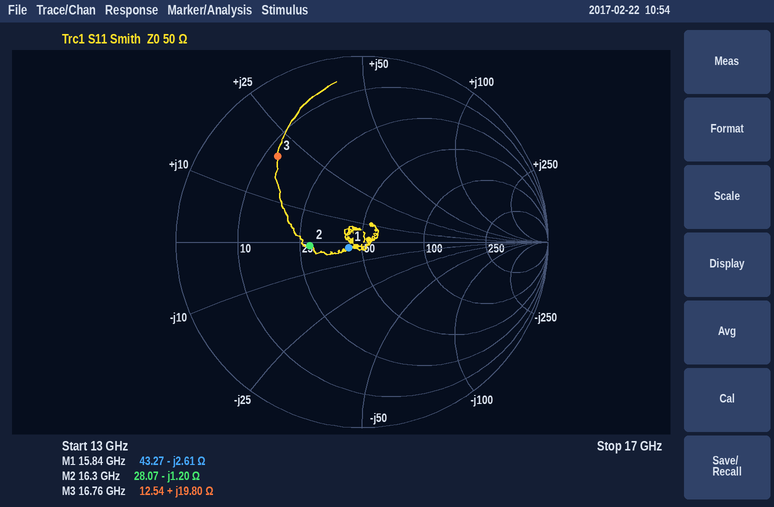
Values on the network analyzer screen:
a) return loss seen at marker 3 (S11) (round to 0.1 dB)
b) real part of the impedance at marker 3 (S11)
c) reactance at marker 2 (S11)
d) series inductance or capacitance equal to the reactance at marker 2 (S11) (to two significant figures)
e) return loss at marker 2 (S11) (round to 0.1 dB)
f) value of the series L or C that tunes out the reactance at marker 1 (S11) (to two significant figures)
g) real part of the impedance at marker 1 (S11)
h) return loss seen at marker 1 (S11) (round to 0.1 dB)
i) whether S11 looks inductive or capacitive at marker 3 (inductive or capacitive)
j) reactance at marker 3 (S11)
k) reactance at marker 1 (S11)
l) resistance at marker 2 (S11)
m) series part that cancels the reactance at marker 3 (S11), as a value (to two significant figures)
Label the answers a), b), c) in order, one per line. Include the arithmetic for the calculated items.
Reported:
a) 3.8 dB
b) 12.54 Ω
c) -1.20 Ω
d) C = 1/(2π × 16.3 GHz × 1.2 Ω) ≈ 8.1 pF
e) 11.0 dB
f) L = 2.61 Ω/(2π × 15.84 GHz) ≈ 26 pH
g) 43.27 Ω
h) 22.2 dB
i) inductive
j) +19.80 Ω
k) -2.61 Ω
l) 28.07 Ω
m) C = 1/(2π × 16.76 GHz × 19.8 Ω) ≈ 480 fF
